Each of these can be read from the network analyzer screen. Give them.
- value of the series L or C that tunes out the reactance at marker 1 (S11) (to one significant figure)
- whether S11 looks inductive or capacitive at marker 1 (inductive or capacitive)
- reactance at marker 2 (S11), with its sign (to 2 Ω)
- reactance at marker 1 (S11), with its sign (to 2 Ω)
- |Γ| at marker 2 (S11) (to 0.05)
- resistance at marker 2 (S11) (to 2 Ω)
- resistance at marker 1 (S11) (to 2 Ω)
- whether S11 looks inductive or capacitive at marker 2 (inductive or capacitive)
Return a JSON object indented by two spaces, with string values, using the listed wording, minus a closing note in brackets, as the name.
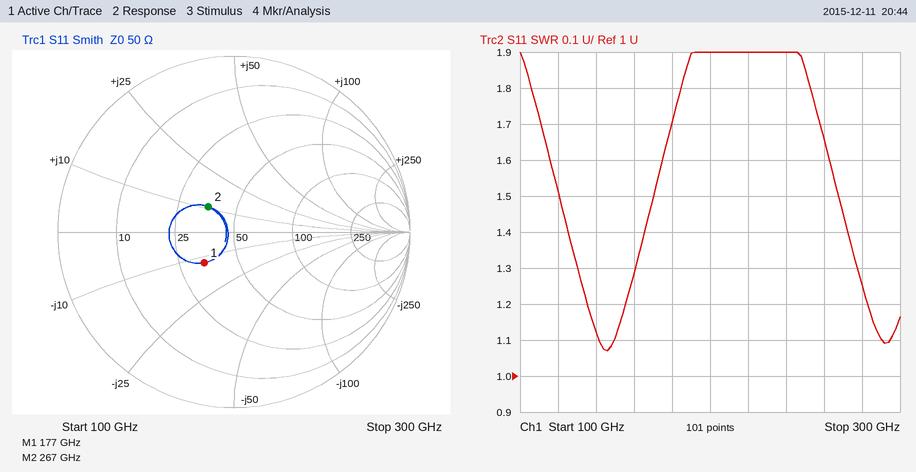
{
  "value of the series L or C that tunes out the reactance at marker 1 (S11)": "10 pH",
  "whether S11 looks inductive or capacitive at marker 1": "capacitive",
  "reactance at marker 2 (S11), with its sign": "+10 Ω",
  "reactance at marker 1 (S11), with its sign": "-12 Ω",
  "|Γ| at marker 2 (S11)": "0.20",
  "resistance at marker 2 (S11)": "36 Ω",
  "resistance at marker 1 (S11)": "34 Ω",
  "whether S11 looks inductive or capacitive at marker 2": "inductive"
}
